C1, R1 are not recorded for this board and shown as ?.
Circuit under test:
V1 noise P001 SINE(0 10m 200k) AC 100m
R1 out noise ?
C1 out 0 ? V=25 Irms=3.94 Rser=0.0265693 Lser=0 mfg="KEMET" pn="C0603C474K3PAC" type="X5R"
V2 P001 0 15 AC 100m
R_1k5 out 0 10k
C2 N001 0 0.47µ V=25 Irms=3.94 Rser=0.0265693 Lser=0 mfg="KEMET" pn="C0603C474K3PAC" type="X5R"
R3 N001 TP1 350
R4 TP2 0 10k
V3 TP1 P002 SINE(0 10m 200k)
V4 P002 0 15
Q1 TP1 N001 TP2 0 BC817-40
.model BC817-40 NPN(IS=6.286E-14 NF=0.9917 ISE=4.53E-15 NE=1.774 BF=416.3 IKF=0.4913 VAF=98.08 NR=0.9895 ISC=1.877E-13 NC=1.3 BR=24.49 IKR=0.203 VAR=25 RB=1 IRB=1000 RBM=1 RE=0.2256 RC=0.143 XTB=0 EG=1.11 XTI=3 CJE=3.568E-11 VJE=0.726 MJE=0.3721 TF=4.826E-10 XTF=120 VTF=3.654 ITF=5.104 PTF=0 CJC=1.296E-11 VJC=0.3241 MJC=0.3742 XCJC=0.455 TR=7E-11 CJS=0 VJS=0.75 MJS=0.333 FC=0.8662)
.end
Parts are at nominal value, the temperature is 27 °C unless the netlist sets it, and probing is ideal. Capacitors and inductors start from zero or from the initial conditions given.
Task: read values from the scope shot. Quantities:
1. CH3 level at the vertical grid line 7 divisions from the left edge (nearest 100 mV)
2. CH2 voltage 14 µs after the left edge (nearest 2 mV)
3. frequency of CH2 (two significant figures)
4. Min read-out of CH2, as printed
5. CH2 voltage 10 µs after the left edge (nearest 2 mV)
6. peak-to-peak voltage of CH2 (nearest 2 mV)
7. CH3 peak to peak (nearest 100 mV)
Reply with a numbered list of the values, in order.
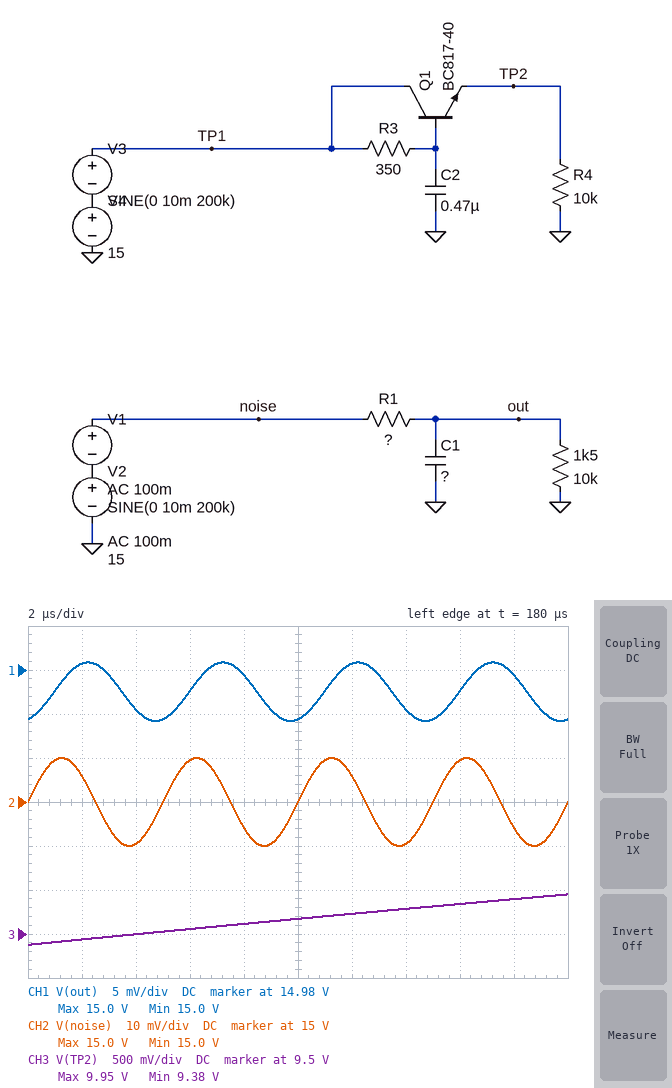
1. 9.8 V
2. 14.990 V
3. 200 kHz
4. 15.0 V
5. 15.000 V
6. 20 mV
7. 600 mV
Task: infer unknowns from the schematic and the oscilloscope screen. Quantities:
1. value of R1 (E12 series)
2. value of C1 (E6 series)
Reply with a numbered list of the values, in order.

1. 15 Ω
2. 150 nF
